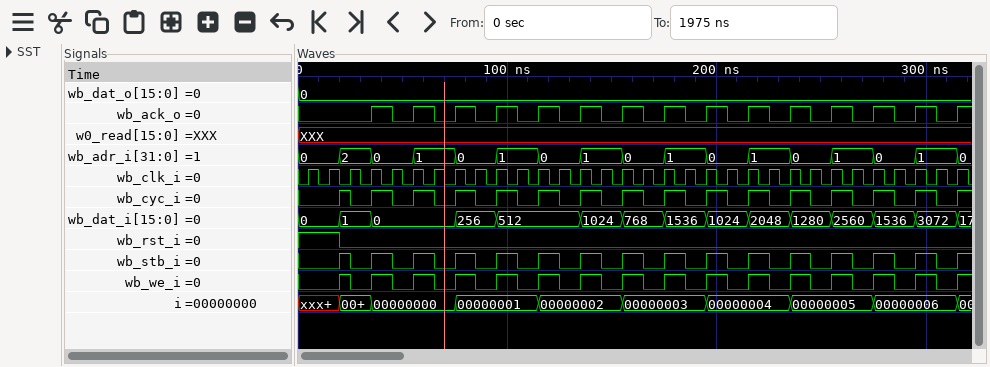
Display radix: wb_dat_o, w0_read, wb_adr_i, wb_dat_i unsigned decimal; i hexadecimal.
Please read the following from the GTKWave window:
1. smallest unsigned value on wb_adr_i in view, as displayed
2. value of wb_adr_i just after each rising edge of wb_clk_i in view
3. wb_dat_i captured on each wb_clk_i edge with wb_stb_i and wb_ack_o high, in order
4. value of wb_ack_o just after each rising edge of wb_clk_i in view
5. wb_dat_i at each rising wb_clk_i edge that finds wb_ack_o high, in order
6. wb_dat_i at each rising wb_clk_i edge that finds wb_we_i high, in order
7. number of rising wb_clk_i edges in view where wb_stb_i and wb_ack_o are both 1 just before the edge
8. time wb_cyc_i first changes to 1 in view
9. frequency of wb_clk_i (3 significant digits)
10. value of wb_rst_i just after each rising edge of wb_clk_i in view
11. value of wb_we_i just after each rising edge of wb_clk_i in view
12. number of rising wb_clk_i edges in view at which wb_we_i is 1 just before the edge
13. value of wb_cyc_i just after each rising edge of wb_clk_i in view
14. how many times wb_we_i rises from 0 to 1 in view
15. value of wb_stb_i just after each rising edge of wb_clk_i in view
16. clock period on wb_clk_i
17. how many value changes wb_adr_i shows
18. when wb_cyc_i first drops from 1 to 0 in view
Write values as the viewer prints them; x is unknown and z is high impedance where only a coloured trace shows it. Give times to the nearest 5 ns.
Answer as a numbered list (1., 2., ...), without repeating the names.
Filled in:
1. 0
2. 0, 0, 2, 0, 0, 1, 1, 0, 0, 1, 1, 0, 0, 1, 1, 0, 0, 1, 1, 0, 0, 1, 1, 0, 0, 1, 1, 0, 0, 1, 1, 0
3. 0, 0, 256, 512, 512, 1024, 768, 1536, 1024, 2048, 1280, 2560, 1536, 3072
4. 0 0 0 1 0 1 0 1 0 1 0 1 0 1 0 1 0 1 0 1 0 1 0 1 0 1 0 1 0 1 0 1
5. 0, 0, 256, 512, 512, 1024, 768, 1536, 1024, 2048, 1280, 2560, 1536, 3072
6. 1, 0, 0, 256, 512, 512, 1024, 768, 1536, 1024, 2048, 1280, 2560, 1536, 3072
7. 14
8. 20 ns
9. 100 MHz
10. 1 1 0 0 0 0 0 0 0 0 0 0 0 0 0 0 0 0 0 0 0 0 0 0 0 0 0 0 0 0 0 0
11. 0 0 0 1 0 1 0 1 0 1 0 1 0 1 0 1 0 1 0 1 0 1 0 1 0 1 0 1 0 1 0 1
12. 15
13. 0 0 0 1 0 1 0 1 0 1 0 1 0 1 0 1 0 1 0 1 0 1 0 1 0 1 0 1 0 1 0 1
14. 16
15. 0 0 0 1 0 1 0 1 0 1 0 1 0 1 0 1 0 1 0 1 0 1 0 1 0 1 0 1 0 1 0 1
16. 10 ns
17. 16
18. 25 ns
